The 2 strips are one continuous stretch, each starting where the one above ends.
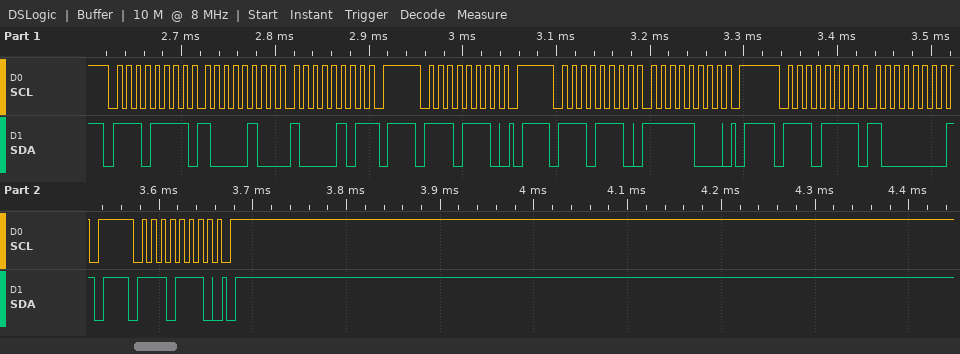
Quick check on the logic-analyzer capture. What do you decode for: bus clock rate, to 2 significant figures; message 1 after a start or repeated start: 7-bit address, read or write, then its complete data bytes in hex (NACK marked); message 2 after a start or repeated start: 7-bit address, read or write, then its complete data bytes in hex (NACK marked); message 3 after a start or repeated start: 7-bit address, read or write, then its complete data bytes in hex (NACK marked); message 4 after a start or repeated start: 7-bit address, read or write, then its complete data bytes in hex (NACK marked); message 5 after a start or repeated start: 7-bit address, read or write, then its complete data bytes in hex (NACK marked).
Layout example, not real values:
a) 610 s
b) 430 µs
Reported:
a) 100 kHz
b) 0x77 read: 84 85 NACK
c) 0x77 write
d) 0x77 write: F8
e) 0x77 read: 80 NACK
f) 0x77 write
